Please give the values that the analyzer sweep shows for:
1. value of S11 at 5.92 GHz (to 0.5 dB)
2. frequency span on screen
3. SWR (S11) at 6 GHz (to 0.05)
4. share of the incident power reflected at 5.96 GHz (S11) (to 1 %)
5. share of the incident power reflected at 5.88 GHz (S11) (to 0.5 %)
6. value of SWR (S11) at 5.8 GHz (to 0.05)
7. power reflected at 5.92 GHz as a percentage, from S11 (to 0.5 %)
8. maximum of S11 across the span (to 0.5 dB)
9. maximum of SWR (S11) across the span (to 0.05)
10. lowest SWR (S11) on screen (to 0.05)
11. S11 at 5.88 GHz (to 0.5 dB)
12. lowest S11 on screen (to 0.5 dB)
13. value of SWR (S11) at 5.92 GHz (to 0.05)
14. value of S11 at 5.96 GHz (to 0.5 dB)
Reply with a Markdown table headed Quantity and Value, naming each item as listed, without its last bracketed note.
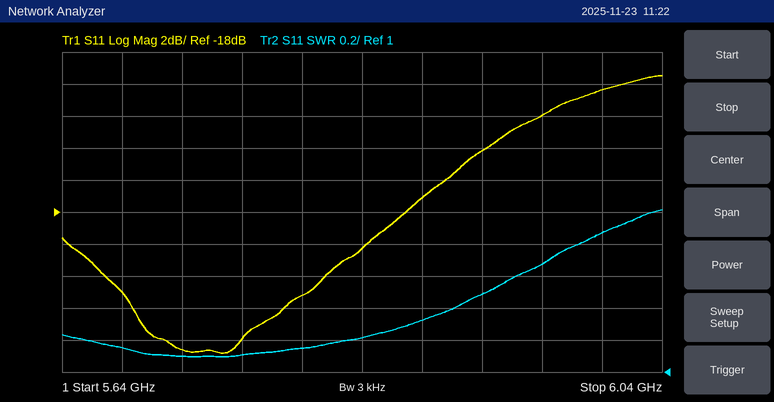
| Quantity | Value |
|---|---|
| value of S11 at 5.92 GHz | -14.0 dB |
| frequency span on screen | 400 MHz |
| SWR (S11) at 6 GHz | 1.85 |
| share of the incident power reflected at 5.96 GHz (S11) | 6 % |
| share of the incident power reflected at 5.88 GHz (S11) | 2.0 % |
| value of SWR (S11) at 5.8 GHz | 1.15 |
| power reflected at 5.92 GHz as a percentage, from S11 | 4.0 % |
| maximum of S11 across the span | -9.5 dB |
| maximum of SWR (S11) across the span | 2.00 |
| lowest SWR (S11) on screen | 1.10 |
| S11 at 5.88 GHz | -17.0 dB |
| lowest S11 on screen | -27.0 dB |
| value of SWR (S11) at 5.92 GHz | 1.50 |
| value of S11 at 5.96 GHz | -12.0 dB |
